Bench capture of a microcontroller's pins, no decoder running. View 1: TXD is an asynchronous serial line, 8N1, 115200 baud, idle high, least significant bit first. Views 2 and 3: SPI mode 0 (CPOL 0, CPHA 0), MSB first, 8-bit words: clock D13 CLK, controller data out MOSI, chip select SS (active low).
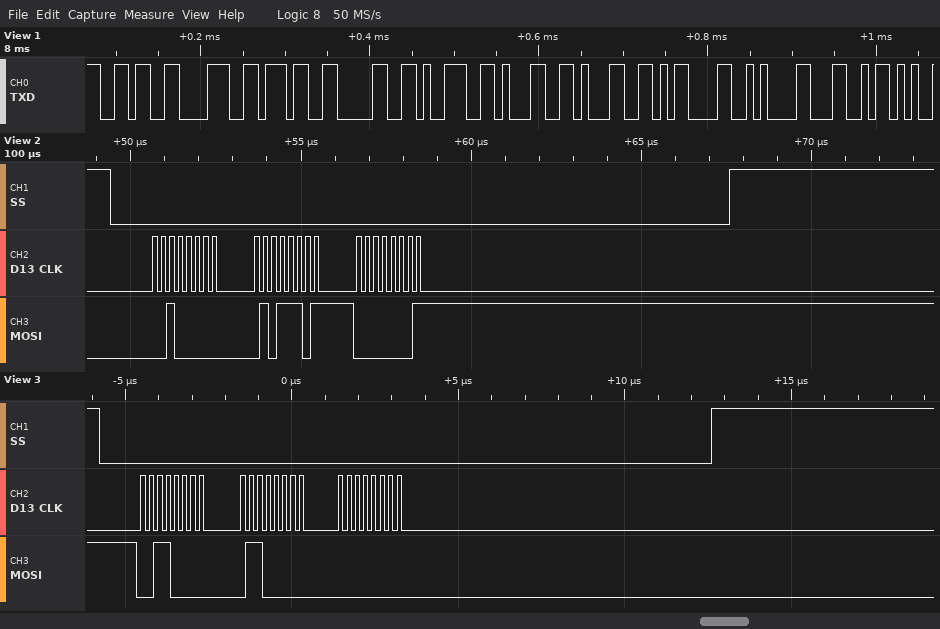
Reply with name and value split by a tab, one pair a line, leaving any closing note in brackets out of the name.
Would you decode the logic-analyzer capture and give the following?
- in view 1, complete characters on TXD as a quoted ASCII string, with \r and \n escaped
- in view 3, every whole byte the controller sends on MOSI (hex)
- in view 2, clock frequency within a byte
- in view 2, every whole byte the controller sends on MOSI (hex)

in view 1, complete characters on TXD as a quoted ASCII string, with \r and \n escaped	"6870911\r\nL"
in view 3, every whole byte the controller sends on MOSI	0x30 0x60 0x00
in view 2, clock frequency within a byte	4 MHz
in view 2, every whole byte the controller sends on MOSI	20 5D 01
